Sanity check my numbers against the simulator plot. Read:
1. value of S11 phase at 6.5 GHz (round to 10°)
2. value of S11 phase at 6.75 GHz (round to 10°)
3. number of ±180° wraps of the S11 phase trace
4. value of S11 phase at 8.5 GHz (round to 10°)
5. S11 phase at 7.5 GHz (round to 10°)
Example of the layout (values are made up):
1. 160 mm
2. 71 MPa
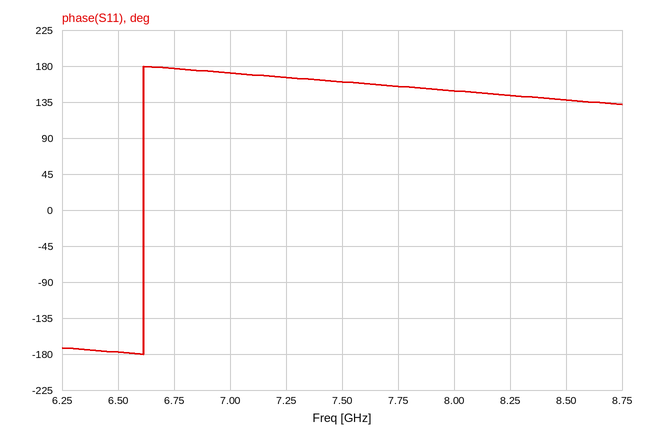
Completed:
1. -180°
2. 180°
3. 1
4. 140°
5. 160°
